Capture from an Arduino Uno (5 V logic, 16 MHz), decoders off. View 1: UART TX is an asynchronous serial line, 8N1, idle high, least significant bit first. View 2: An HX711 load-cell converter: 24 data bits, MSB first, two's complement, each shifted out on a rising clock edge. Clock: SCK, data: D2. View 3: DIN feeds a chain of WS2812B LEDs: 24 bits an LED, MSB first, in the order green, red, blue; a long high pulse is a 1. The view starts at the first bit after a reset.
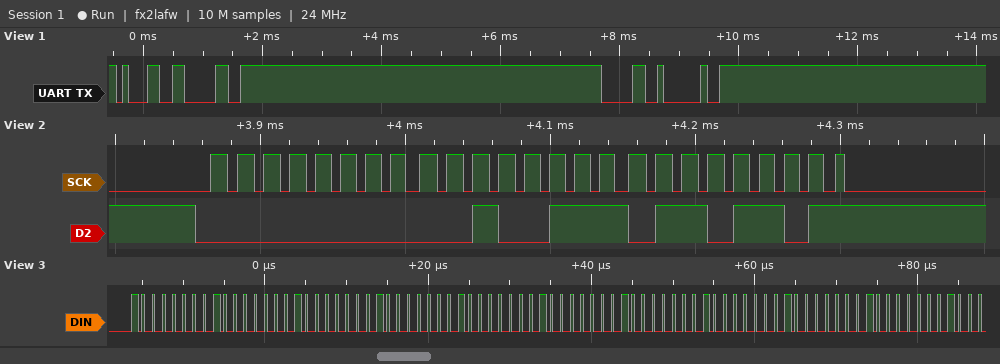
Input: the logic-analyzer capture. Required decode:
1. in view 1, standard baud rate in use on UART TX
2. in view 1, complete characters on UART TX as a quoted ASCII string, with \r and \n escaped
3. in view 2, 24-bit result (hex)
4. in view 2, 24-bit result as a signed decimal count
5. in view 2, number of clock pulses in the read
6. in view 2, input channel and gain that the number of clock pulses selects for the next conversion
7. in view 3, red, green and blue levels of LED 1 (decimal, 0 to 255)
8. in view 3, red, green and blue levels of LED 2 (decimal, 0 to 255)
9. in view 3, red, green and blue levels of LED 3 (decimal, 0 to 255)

9600 baud
"100 "
0x00276D
10093
25
channel A, gain 128
128, 128, 128
128, 128, 128
128, 128, 128
